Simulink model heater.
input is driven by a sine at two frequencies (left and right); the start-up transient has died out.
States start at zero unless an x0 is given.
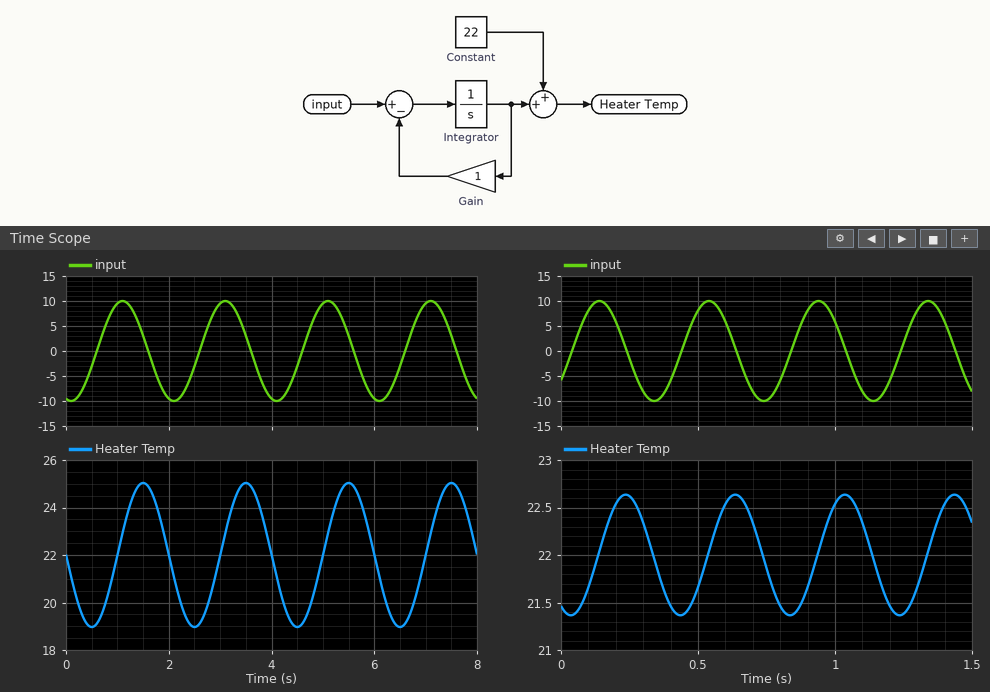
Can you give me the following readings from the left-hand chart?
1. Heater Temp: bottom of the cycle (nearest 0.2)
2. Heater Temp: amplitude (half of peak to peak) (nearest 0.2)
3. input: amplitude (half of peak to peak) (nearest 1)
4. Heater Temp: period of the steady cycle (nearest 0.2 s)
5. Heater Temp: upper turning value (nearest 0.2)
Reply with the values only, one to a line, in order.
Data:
19.0
3.0
10
2.0 s
25.0
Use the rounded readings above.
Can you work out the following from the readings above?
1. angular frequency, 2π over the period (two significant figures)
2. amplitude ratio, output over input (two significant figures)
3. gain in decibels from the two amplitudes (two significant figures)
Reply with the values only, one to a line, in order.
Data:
3.1 rad/s
0.30
-10 dB
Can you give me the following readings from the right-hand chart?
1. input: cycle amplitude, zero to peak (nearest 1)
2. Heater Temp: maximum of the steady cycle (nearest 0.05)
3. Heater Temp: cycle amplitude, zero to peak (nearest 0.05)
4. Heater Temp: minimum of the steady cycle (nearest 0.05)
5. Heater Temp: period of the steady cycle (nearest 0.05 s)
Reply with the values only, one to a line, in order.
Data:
10
22.65
0.65
21.35
0.40 s
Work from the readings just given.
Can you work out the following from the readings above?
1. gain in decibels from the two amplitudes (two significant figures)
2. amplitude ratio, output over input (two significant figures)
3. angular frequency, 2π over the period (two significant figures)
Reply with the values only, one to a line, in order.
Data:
-24 dB
0.065
16 rad/s
